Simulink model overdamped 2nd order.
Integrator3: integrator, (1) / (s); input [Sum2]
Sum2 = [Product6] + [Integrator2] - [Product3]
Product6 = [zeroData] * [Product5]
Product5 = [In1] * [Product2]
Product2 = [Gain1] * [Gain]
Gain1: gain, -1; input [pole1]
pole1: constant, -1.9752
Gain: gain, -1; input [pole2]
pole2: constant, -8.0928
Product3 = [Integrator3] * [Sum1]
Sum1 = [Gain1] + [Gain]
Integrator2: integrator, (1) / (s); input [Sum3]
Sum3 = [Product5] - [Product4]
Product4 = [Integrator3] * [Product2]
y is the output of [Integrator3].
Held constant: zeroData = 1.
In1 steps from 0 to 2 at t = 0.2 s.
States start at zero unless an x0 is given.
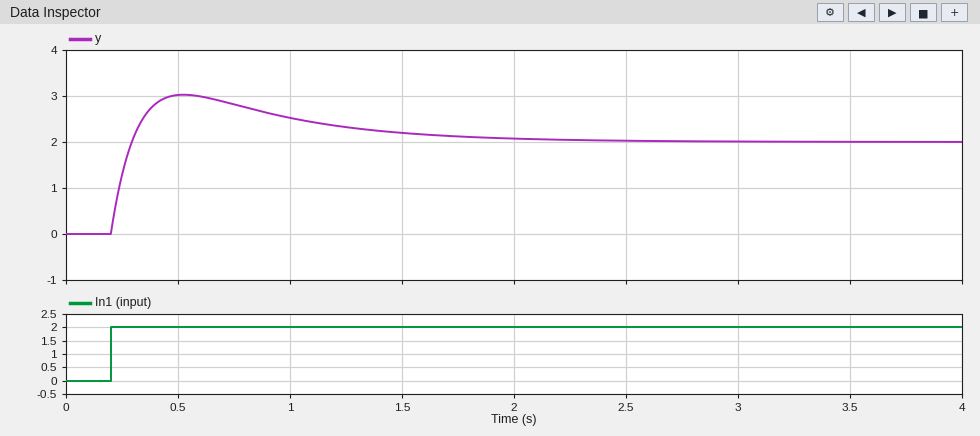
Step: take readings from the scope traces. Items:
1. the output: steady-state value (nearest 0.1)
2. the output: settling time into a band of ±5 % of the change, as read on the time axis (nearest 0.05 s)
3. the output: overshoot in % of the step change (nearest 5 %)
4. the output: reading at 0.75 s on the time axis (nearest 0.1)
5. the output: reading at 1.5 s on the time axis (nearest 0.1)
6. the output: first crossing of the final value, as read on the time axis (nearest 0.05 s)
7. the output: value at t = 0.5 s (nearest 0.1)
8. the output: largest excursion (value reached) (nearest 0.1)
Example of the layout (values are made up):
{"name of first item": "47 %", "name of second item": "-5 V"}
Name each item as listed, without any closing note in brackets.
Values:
{"the output: steady-state value": "2.0", "the output: settling time into a band of ±5 % of the change, as read on the time axis": "1.85 s", "the output: overshoot in % of the step change": "50 %", "the output: reading at 0.75 s on the time axis": "2.8", "the output: reading at 1.5 s on the time axis": "2.2", "the output: first crossing of the final value, as read on the time axis": "0.30 s", "the output: value at t = 0.5 s": "3.0", "the output: largest excursion (value reached)": "3.0"}
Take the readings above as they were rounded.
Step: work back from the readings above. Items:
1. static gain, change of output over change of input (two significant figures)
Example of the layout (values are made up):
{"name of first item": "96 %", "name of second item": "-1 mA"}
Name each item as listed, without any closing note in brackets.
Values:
{"static gain, change of output over change of input": "1.0"}
